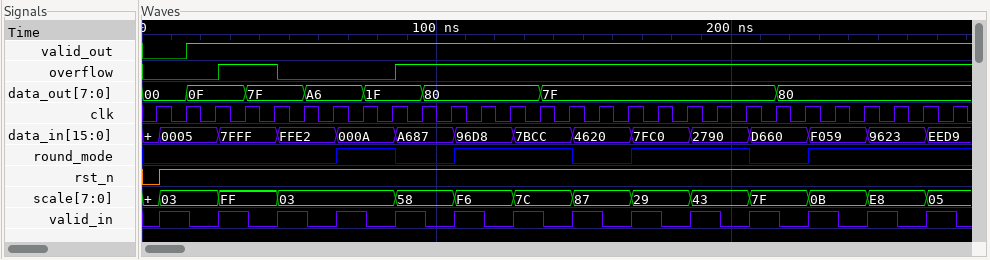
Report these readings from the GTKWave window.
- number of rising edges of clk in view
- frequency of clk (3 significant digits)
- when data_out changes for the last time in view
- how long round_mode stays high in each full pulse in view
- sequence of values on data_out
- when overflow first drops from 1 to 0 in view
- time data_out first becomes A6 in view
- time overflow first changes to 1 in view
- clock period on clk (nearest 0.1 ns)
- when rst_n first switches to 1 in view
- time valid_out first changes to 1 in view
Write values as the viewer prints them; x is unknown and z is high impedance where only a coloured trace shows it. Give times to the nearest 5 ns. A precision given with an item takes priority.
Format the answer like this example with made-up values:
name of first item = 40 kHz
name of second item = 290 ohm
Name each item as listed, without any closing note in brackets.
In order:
number of rising edges of clk in view = 28
frequency of clk = 100 MHz
when data_out changes for the last time in view = 215 ns
how long round_mode stays high in each full pulse in view = 20 ns, 40 ns, 40 ns
sequence of values on data_out = 00, 0F, 7F, A6, 1F, 80, 7F, 80
when overflow first drops from 1 to 0 in view = 45 ns
time data_out first becomes A6 in view = 55 ns
time overflow first changes to 1 in view = 25 ns
clock period on clk = 10 ns
when rst_n first switches to 1 in view = 5 ns
time valid_out first changes to 1 in view = 15 ns
